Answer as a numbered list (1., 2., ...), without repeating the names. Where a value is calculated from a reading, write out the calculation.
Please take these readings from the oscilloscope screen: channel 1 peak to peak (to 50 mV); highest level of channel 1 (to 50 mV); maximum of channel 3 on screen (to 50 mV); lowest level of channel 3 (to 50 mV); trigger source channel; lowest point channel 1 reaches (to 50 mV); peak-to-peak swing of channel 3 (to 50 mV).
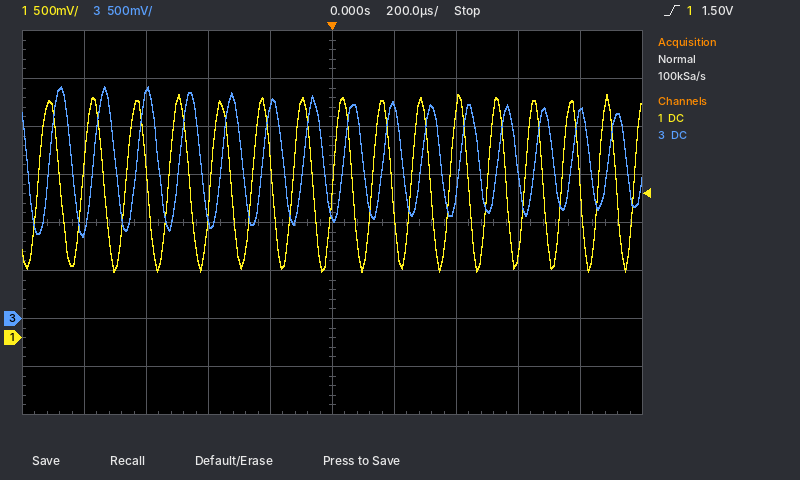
1. 2.55 V − (700 mV) = 1.85 V
2. 2.55 V
3. 2.40 V
4. 850 mV
5. channel 1
6. 700 mV
7. 2.40 V − (850 mV) = 1.55 V
